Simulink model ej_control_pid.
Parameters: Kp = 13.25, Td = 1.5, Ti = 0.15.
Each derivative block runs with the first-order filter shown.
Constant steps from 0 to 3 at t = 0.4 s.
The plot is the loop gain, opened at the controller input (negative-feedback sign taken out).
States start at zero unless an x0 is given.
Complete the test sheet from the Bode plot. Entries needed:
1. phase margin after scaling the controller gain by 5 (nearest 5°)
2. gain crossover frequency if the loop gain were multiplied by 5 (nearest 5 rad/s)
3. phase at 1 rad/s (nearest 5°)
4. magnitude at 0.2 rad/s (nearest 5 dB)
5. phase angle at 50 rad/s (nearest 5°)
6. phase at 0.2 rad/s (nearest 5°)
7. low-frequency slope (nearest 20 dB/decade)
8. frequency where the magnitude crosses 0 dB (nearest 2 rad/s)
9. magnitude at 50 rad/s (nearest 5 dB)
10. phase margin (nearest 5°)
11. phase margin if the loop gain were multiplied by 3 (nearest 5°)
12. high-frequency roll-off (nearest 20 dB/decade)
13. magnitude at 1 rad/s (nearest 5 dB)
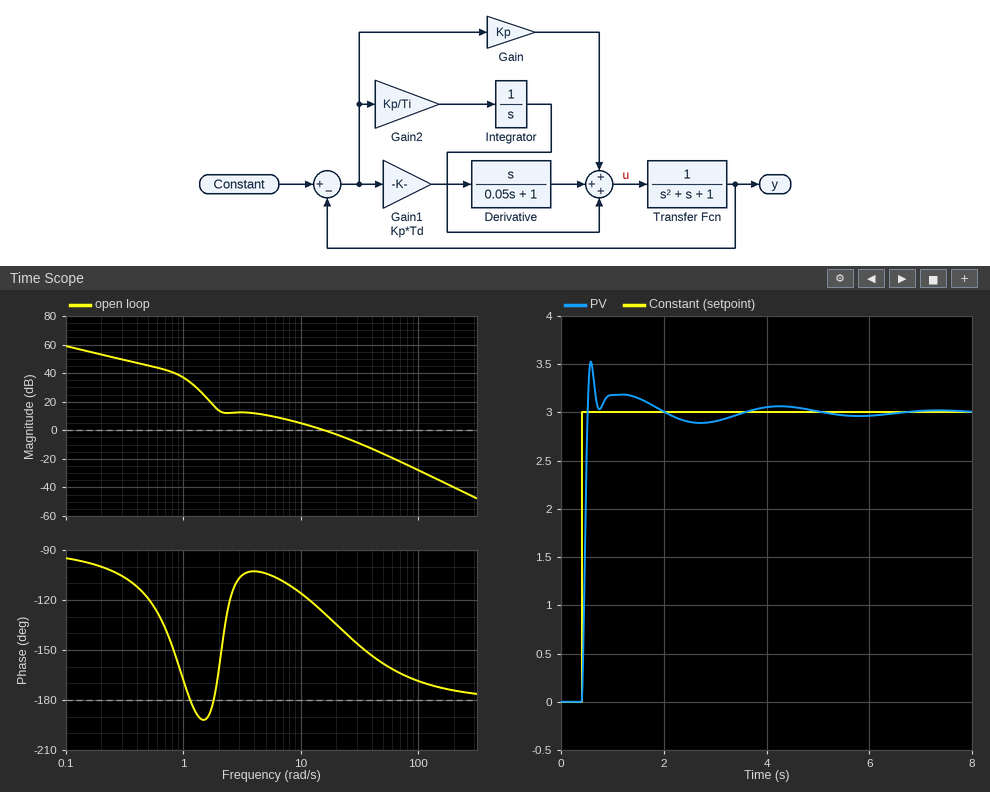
25°
45 rad/s
-170°
55 dB
-160°
-100°
-20 dB/decade
16 rad/s
-15 dB
50°
30°
-40 dB/decade
35 dB
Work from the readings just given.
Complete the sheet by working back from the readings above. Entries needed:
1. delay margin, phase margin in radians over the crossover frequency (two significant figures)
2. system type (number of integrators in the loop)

0.055 s
1
